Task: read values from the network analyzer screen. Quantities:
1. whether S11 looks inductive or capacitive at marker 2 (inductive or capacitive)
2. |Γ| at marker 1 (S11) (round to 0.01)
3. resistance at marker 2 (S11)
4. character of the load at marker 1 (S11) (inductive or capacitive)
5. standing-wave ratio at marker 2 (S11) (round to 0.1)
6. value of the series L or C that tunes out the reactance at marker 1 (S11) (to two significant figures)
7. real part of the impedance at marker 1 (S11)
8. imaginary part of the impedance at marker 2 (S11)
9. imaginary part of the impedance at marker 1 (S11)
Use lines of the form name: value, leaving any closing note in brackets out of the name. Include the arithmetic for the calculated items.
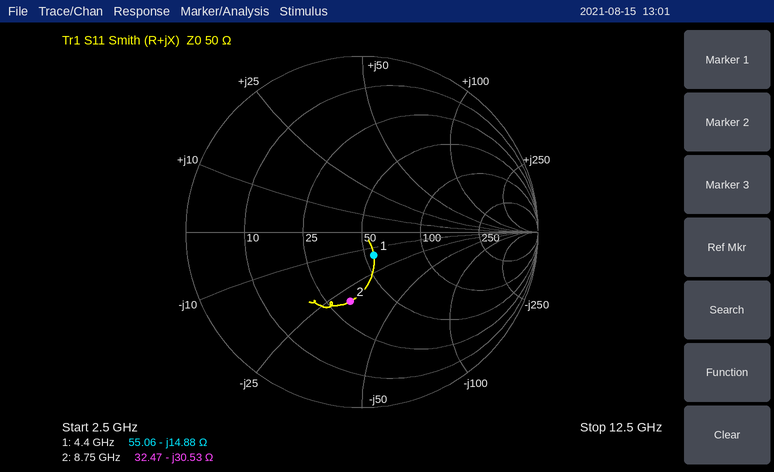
whether S11 looks inductive or capacitive at marker 2: capacitive
|Γ| at marker 1 (S11): 0.15
resistance at marker 2: 32.47 Ω
character of the load at marker 1 (S11): capacitive
standing-wave ratio at marker 2 (S11): 2.3
value of the series L or C that tunes out the reactance at marker 1 (S11): L = 14.88 Ω/(2π × 4.4 GHz) ≈ 538 pH, so 540 pH to two significant figures
real part of the impedance at marker 1: 55.06 Ω
imaginary part of the impedance at marker 2: -30.53 Ω
imaginary part of the impedance at marker 1: -14.88 Ω
